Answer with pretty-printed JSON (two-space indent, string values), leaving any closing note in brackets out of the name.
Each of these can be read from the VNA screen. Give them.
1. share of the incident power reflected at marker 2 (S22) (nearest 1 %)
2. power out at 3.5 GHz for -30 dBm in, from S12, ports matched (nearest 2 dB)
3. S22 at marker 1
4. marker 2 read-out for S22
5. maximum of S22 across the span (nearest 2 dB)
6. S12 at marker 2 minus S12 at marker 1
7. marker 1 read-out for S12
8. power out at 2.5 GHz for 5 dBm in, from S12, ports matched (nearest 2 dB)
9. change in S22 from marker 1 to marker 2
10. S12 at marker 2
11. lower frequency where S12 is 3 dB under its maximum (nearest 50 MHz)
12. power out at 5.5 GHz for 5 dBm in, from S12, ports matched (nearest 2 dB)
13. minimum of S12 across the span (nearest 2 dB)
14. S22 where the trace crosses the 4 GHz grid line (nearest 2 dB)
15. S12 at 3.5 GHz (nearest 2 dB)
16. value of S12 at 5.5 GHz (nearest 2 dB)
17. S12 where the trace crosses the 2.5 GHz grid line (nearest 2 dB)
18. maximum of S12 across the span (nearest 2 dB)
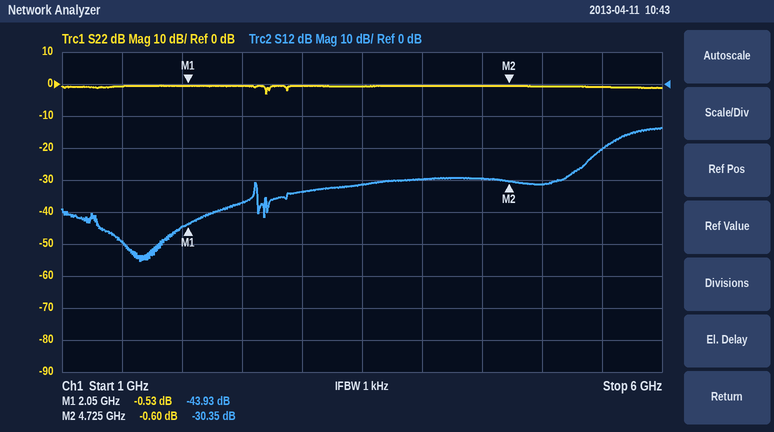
{
  "share of the incident power reflected at marker 2 (S22)": "87 %",
  "power out at 3.5 GHz for -30 dBm in, from S12, ports matched": "-62 dBm",
  "S22 at marker 1": "-0.53 dB",
  "marker 2 read-out for S22": "-0.60 dB",
  "maximum of S22 across the span": "0 dB",
  "S12 at marker 2 minus S12 at marker 1": "13.58 dB",
  "marker 1 read-out for S12": "-43.93 dB",
  "power out at 2.5 GHz for 5 dBm in, from S12, ports matched": "-32 dBm",
  "change in S22 from marker 1 to marker 2": "-0.07 dB",
  "S12 at marker 2": "-30.35 dB",
  "lower frequency where S12 is 3 dB under its maximum": "5.65 GHz",
  "power out at 5.5 GHz for 5 dBm in, from S12, ports matched": "-16 dBm",
  "minimum of S12 across the span": "-56 dB",
  "S22 where the trace crosses the 4 GHz grid line": "0 dB",
  "S12 at 3.5 GHz": "-32 dB",
  "value of S12 at 5.5 GHz": "-20 dB",
  "S12 where the trace crosses the 2.5 GHz grid line": "-38 dB",
  "maximum of S12 across the span": "-14 dB"
}
